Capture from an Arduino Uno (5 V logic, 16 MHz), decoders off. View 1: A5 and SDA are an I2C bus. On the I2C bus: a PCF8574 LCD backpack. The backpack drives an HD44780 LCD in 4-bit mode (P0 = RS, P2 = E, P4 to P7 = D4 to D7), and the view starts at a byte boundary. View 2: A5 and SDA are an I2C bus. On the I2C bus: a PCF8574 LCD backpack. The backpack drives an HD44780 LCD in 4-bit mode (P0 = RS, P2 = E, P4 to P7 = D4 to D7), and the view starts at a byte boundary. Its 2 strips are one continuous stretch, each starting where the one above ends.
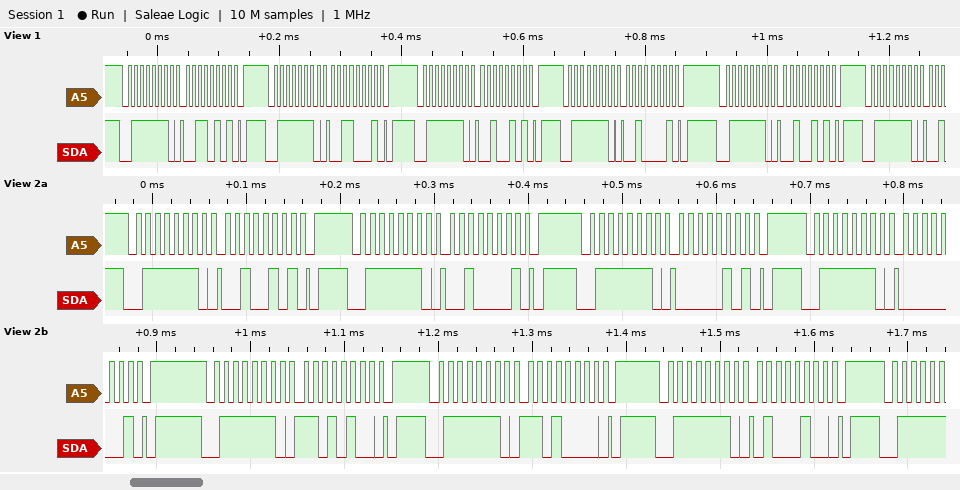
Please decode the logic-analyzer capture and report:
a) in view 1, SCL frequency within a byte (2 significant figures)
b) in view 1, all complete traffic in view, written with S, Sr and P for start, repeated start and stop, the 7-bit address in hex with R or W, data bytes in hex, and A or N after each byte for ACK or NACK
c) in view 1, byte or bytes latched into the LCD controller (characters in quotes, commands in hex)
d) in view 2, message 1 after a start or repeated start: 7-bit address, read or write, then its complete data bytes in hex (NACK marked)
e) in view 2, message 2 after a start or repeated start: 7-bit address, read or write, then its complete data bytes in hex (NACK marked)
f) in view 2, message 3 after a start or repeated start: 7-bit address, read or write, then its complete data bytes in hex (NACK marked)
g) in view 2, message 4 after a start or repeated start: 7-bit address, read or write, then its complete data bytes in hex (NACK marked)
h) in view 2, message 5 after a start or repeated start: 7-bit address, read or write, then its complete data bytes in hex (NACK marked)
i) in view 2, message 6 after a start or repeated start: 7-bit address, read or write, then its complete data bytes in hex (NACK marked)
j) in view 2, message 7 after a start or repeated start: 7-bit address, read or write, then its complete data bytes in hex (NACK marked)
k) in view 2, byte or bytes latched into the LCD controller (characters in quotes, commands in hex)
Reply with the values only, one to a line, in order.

100 kHz
S 3FW A 35 A P S 3FW A 31 A P S 3FW A 25 A P S 3FW A 21 A P S 3FW A 25 A P S 3FW A
'2'
0x3F write: 25
0x3F write: 21
0x3F write: 05
0x3F write: 01
0x3F write: D4
0x3F write: D0
0x3F write: 44
' '
